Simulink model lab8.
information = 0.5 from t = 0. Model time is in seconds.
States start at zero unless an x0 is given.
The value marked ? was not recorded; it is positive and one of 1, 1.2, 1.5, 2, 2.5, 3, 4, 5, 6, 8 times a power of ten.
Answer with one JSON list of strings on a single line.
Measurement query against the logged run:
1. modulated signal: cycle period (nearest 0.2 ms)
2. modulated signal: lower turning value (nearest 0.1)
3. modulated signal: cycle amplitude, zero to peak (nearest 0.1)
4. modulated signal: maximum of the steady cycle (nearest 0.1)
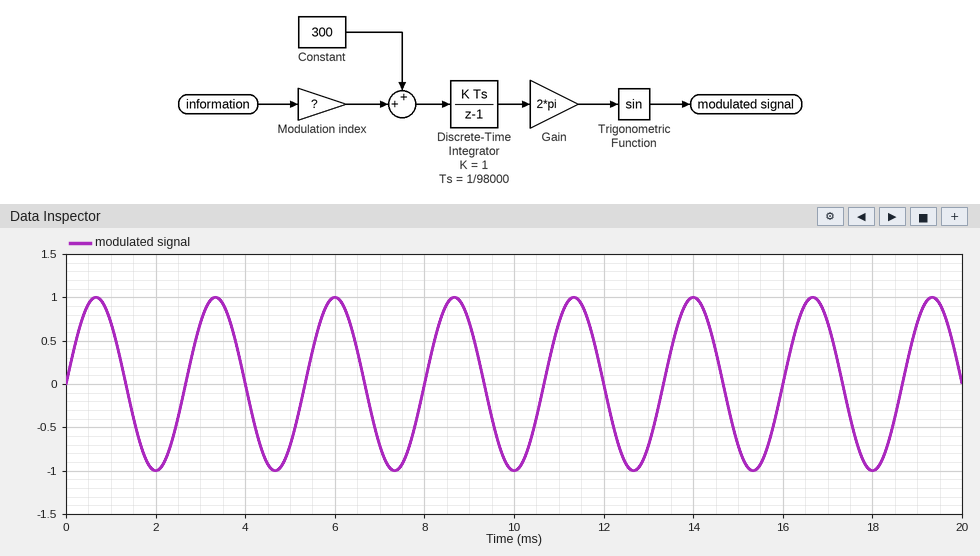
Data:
["2.6 ms", "-1.0", "1.0", "1.0"]
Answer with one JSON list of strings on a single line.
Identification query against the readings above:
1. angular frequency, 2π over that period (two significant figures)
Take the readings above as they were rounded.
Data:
["2.4 rad/ms"]
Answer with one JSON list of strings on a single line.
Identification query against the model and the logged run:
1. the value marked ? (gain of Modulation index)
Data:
["150"]
